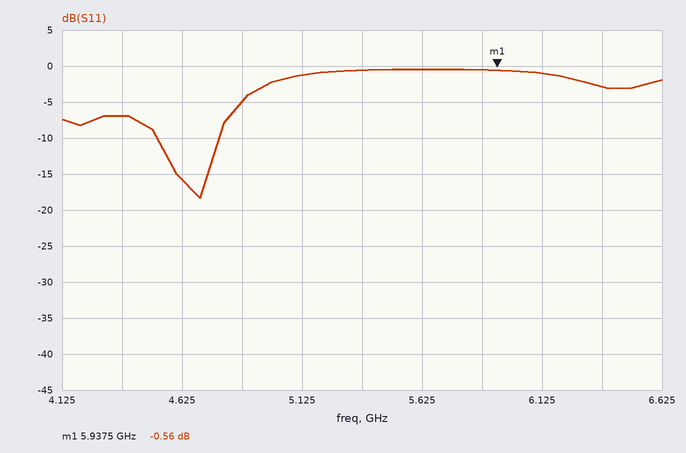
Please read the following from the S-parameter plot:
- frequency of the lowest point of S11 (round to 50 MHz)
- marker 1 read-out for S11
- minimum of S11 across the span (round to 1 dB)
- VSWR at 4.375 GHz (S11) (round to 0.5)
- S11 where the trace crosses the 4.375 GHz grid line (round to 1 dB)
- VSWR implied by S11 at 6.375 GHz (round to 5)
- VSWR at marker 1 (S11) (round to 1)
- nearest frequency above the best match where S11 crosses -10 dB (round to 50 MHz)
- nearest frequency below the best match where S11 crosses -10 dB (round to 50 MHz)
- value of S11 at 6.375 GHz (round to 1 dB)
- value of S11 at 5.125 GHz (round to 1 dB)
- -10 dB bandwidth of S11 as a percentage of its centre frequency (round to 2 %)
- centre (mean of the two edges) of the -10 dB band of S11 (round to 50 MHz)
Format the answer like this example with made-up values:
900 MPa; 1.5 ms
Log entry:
4.70 GHz; -0.56 dB; -18 dB; 2.5; -7 dB; 5; 31; 4.80 GHz; 4.50 GHz; -3 dB; -1 dB; 6 %; 4.65 GHz
